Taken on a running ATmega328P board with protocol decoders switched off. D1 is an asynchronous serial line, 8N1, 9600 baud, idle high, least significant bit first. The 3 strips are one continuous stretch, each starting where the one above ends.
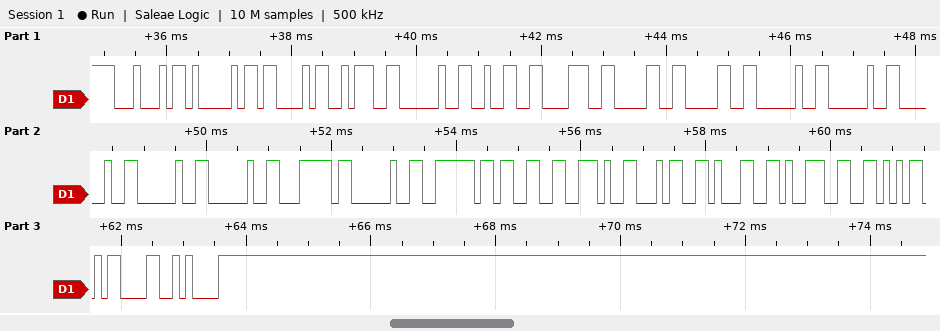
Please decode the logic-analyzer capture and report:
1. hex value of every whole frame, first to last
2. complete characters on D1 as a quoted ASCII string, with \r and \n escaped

44 41 43 3A 20 32 38 30 30 20 20 20 20 20 7C 20 7E 33 2E 34 31 39 56 0D 0A
"DAC: 2800     | ~3.419V\r\n"
